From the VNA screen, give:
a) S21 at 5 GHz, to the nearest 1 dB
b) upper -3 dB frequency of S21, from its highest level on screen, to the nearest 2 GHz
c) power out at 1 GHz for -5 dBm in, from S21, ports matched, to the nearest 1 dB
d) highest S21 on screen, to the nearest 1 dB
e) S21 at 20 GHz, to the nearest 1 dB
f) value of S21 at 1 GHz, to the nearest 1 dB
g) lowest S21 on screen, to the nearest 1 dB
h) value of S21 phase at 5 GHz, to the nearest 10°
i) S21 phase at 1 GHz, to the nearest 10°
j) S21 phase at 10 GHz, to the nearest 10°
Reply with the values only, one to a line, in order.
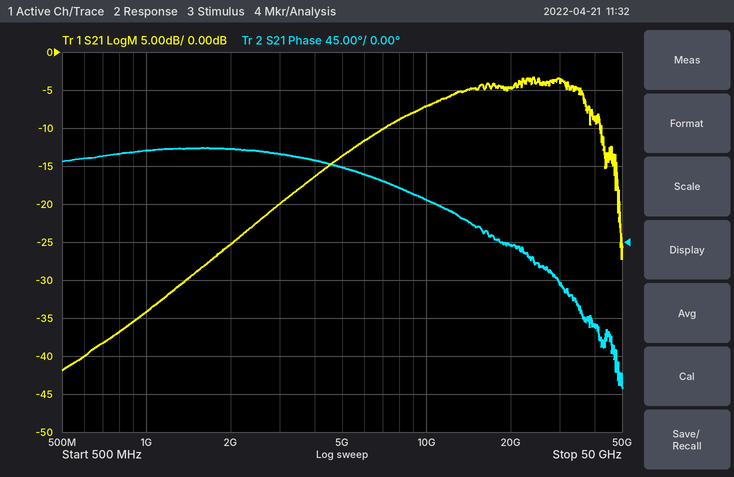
-14 dB
36 GHz
-39 dBm
-3 dB
-5 dB
-34 dB
-42 dB
90°
110°
50°
